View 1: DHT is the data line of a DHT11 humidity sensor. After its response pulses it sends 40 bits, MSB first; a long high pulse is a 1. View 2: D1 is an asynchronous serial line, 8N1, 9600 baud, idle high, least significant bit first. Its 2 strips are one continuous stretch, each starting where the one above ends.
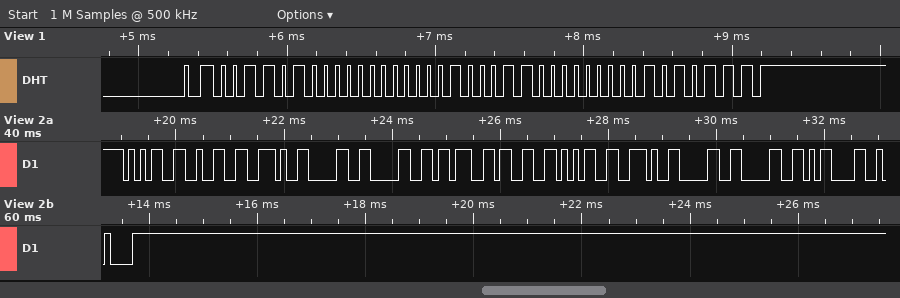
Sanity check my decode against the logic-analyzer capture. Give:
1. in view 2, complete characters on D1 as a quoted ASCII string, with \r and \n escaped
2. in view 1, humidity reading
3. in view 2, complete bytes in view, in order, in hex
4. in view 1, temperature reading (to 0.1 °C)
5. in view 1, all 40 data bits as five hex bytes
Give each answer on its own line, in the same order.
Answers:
"52.00;35.00\r\n"
52 %
0x35 0x32 0x2E 0x30 0x30 0x3B 0x33 0x35 0x2E 0x30 0x30 0x0D 0x0A
35.0 °C
34 00 23 00 57
